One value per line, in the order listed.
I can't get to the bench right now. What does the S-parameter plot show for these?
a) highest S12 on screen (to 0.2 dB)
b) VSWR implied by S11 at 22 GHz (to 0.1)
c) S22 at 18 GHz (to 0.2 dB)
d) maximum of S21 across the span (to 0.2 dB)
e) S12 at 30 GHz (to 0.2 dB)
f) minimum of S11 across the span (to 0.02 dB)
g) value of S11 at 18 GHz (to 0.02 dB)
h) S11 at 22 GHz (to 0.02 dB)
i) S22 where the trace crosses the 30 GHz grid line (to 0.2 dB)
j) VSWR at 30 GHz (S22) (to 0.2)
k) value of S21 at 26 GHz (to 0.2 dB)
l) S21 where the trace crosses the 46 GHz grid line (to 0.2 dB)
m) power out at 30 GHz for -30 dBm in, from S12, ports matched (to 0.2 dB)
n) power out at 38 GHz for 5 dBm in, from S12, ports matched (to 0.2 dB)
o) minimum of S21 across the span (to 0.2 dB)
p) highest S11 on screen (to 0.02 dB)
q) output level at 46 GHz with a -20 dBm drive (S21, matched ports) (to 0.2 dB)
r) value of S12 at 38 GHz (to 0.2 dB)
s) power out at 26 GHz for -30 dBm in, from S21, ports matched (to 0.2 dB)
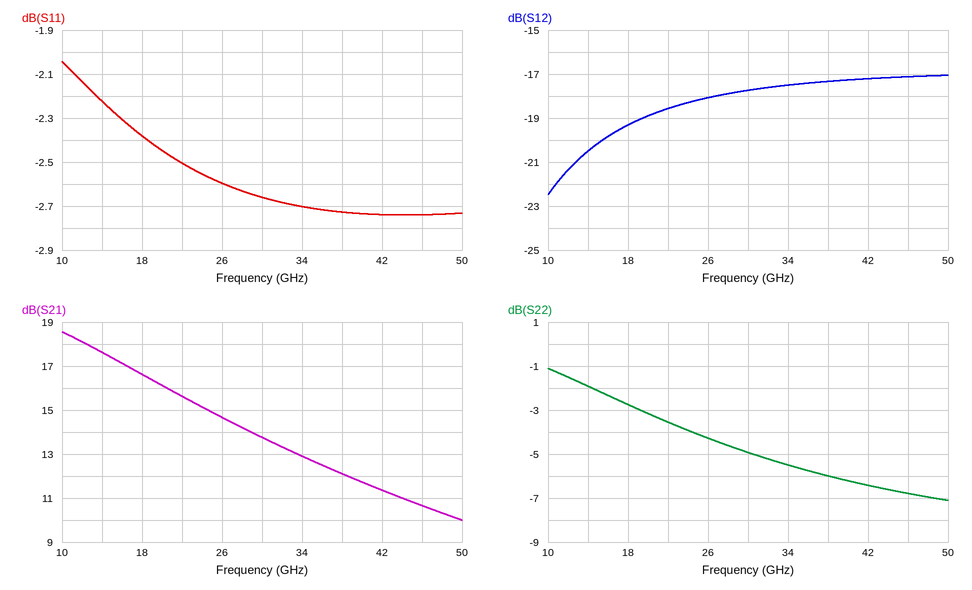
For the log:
-17.0 dB
7.0
-2.8 dB
18.6 dB
-17.8 dB
-2.74 dB
-2.38 dB
-2.50 dB
-5.0 dB
3.6
14.6 dB
10.6 dB
-47.8 dBm
-12.4 dBm
10.0 dB
-2.04 dB
-9.4 dBm
-17.4 dB
-15.4 dBm
